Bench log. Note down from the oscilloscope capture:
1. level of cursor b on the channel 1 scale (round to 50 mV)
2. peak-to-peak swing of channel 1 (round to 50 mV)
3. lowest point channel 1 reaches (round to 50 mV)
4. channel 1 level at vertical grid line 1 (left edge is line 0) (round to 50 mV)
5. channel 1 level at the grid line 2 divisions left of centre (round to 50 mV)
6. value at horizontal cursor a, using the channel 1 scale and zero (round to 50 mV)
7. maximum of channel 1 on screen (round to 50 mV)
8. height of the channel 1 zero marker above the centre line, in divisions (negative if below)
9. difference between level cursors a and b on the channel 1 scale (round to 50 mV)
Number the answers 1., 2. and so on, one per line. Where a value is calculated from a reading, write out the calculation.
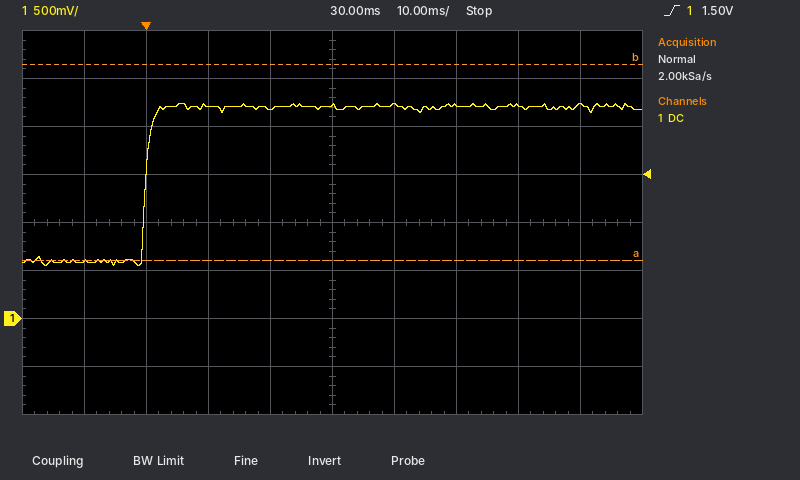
1. 2.65 V
2. 2.25 V − (550 mV) = 1.70 V
3. 550 mV
4. 600 mV
5. 2.20 V
6. 600 mV
7. 2.25 V
8. -2.0 div
9. 2.05 V
